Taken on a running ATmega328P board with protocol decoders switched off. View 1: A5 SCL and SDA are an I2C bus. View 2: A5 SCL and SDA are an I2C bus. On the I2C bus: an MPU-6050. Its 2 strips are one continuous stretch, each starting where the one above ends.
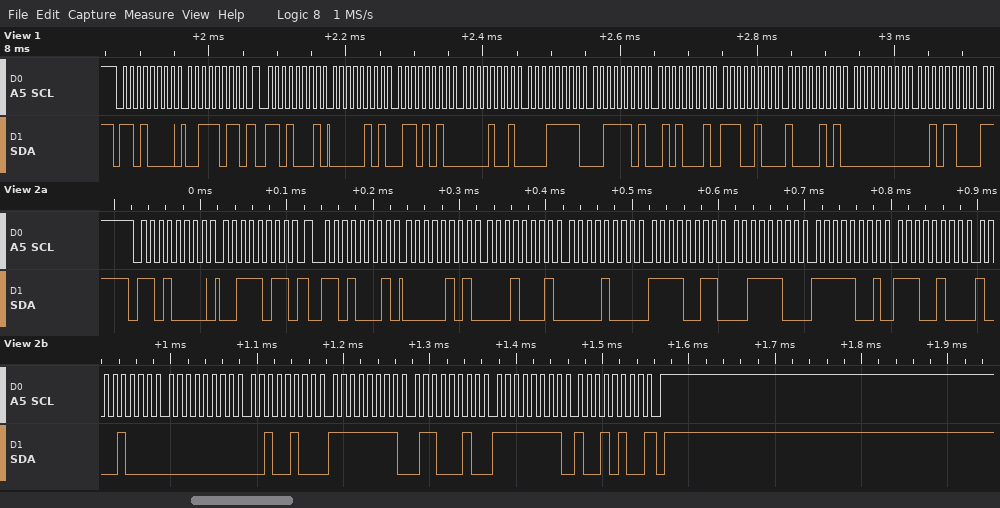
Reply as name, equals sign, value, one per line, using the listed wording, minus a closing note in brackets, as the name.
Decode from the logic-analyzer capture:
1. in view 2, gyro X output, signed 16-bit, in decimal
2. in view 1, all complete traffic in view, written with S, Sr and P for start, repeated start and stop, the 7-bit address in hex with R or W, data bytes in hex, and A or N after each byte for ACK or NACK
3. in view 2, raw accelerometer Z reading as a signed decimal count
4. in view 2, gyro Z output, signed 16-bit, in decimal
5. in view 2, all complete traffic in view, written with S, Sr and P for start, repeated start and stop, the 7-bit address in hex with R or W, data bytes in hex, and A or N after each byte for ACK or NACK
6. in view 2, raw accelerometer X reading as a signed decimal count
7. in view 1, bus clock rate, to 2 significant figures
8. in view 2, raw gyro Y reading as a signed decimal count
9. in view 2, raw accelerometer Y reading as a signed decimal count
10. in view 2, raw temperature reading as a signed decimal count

in view 2, gyro X output, signed 16-bit, in decimal = 36
in view 1, all complete traffic in view, written with S, Sr and P for start, repeated start and stop, the 7-bit address in hex with R or W, data bytes in hex, and A or N after each byte for ACK or NACK = S 68W A 3B A Sr 68R A 05 A 6A A 09 A 1F A 3D A 51 A E4 A 85 A 00 A 2C A
in view 2, raw accelerometer Z reading as a signed decimal count = 15609
in view 2, gyro Z output, signed 16-bit, in decimal = -108
in view 2, all complete traffic in view, written with S, Sr and P for start, repeated start and stop, the 7-bit address in hex with R or W, data bytes in hex, and A or N after each byte for ACK or NACK = S 68W A 3B A Sr 68R A 05 A 11 A 08 A F3 A 3C A F9 A E4 A 88 A 00 A 24 A FF A 62 A FF A 94 N P
in view 2, raw accelerometer X reading as a signed decimal count = 1297
in view 1, bus clock rate, to 2 significant figures = 100 kHz
in view 2, raw gyro Y reading as a signed decimal count = -158
in view 2, raw accelerometer Y reading as a signed decimal count = 2291
in view 2, raw temperature reading as a signed decimal count = -7032
